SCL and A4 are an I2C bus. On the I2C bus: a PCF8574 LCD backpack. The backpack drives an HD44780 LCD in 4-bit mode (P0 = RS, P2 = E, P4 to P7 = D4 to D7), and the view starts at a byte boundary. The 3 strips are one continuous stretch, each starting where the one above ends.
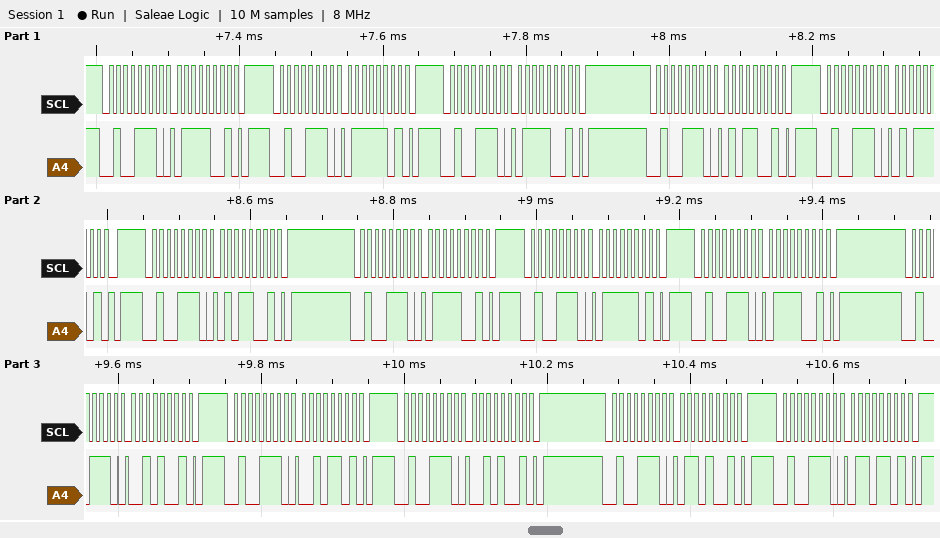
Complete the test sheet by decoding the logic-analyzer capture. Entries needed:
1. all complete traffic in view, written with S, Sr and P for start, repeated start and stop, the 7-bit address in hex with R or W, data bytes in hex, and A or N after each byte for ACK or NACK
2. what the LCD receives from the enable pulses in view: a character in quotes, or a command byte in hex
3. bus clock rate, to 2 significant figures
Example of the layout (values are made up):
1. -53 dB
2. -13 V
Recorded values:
1. S 27W A 79 A P S 27W A 7D A P S 27W A 79 A P S 27W A 59 A P S 27W A 5D A P S 27W A 59 A P S 27W A 79 A P S 27W A 7D A P S 27W A 79 A P S 27W A 29 A P S 27W A 2D A P S 27W A 29 A P S 27W A 69 A P S 27W A 6D A P
2. 'u' 'r'
3. 100 kHz
